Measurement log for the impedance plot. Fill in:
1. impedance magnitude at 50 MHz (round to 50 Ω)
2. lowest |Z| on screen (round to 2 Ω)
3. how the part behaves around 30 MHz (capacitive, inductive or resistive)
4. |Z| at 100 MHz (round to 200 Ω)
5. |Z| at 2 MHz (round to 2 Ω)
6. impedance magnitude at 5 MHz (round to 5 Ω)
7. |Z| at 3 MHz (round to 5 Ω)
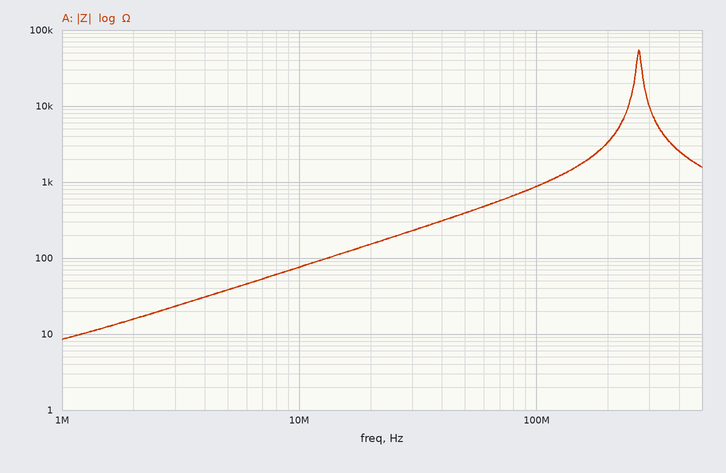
400 Ω
8 Ω
inductive
800 Ω
16 Ω
40 Ω
25 Ω
